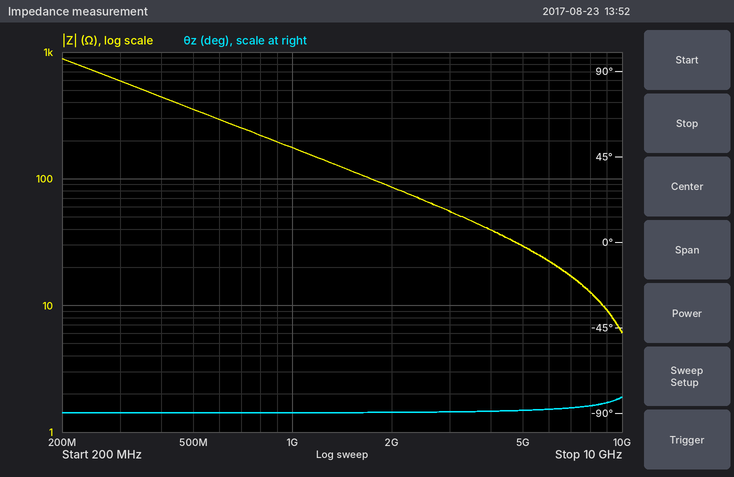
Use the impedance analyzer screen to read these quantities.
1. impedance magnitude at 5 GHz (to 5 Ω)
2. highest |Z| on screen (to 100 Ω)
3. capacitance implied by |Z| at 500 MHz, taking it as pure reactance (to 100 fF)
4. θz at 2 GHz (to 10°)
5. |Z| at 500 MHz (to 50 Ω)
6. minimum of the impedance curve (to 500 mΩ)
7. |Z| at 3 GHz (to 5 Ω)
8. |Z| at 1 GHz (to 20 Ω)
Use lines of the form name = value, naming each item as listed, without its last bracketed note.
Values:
impedance magnitude at 5 GHz = 30 Ω
highest |Z| on screen = 900 Ω
capacitance implied by |Z| at 500 MHz, taking it as pure reactance = 900 fF
θz at 2 GHz = -90°
|Z| at 500 MHz = 350 Ω
minimum of the impedance curve = 6.0 Ω
|Z| at 3 GHz = 55 Ω
|Z| at 1 GHz = 180 Ω
